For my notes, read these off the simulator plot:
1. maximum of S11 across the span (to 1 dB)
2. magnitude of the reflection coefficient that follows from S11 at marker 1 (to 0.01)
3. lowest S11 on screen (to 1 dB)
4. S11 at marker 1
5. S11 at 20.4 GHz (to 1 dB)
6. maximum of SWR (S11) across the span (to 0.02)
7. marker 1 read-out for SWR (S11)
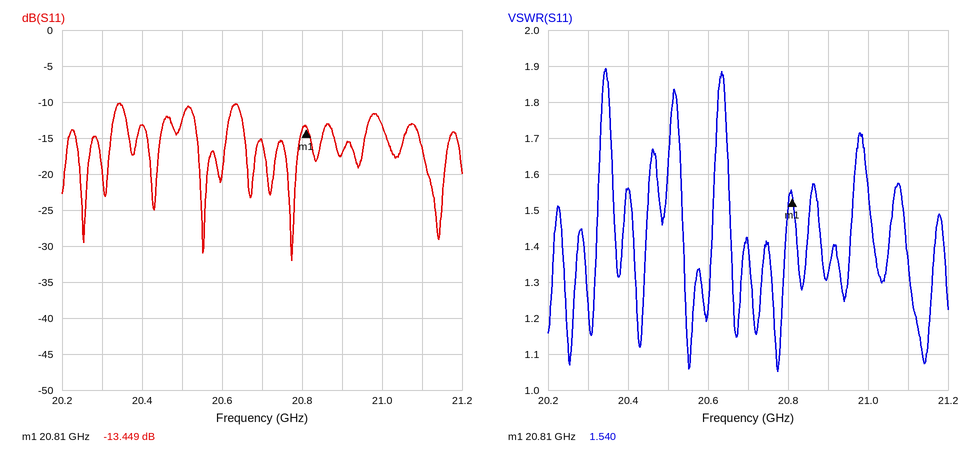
-10 dB
0.21
-32 dB
-13.449 dB
-13 dB
1.90
1.540
